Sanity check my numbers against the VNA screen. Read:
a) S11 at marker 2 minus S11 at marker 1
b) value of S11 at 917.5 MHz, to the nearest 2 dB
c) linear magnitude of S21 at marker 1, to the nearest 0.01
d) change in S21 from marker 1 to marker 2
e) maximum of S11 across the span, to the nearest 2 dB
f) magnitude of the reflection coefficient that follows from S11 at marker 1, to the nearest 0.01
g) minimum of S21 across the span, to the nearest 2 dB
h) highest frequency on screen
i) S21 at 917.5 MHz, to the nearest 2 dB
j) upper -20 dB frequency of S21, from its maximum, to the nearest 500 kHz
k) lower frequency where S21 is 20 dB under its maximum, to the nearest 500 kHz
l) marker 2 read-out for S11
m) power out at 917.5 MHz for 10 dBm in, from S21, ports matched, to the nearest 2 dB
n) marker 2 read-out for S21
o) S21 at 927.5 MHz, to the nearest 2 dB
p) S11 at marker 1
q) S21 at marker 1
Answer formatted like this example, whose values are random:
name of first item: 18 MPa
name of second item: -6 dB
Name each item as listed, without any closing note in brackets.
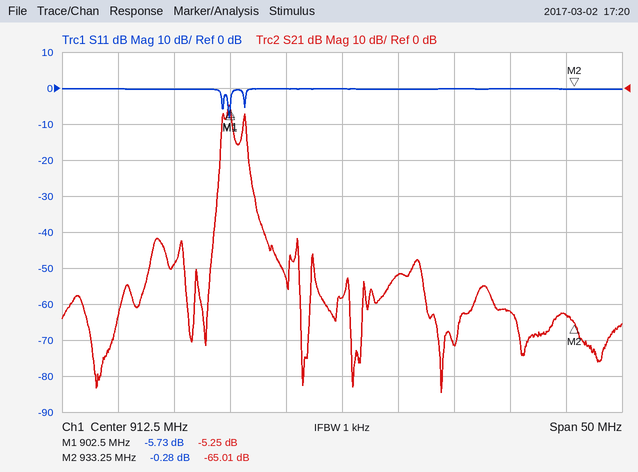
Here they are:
S11 at marker 2 minus S11 at marker 1: 5.45 dB
value of S11 at 917.5 MHz, to the nearest 2 dB: 0 dB
linear magnitude of S21 at marker 1, to the nearest 0.01: 0.55
change in S21 from marker 1 to marker 2: -59.76 dB
maximum of S11 across the span, to the nearest 2 dB: 0 dB
magnitude of the reflection coefficient that follows from S11 at marker 1, to the nearest 0.01: 0.52
minimum of S21 across the span, to the nearest 2 dB: -84 dB
highest frequency on screen: 937.5 MHz
S21 at 917.5 MHz, to the nearest 2 dB: -52 dB
upper -20 dB frequency of S21, from its maximum, to the nearest 500 kHz: 904.5 MHz
lower frequency where S21 is 20 dB under its maximum, to the nearest 500 kHz: 901.5 MHz
marker 2 read-out for S11: -0.28 dB
power out at 917.5 MHz for 10 dBm in, from S21, ports matched, to the nearest 2 dB: -42 dBm
marker 2 read-out for S21: -65.01 dB
S21 at 927.5 MHz, to the nearest 2 dB: -62 dB
S11 at marker 1: -5.73 dB
S21 at marker 1: -5.25 dB
